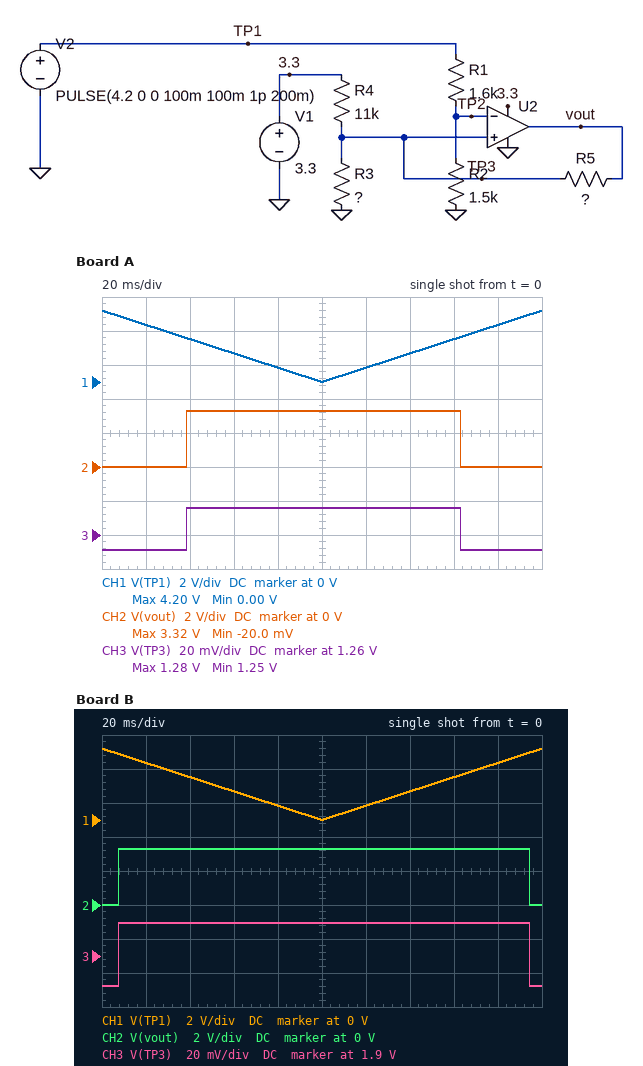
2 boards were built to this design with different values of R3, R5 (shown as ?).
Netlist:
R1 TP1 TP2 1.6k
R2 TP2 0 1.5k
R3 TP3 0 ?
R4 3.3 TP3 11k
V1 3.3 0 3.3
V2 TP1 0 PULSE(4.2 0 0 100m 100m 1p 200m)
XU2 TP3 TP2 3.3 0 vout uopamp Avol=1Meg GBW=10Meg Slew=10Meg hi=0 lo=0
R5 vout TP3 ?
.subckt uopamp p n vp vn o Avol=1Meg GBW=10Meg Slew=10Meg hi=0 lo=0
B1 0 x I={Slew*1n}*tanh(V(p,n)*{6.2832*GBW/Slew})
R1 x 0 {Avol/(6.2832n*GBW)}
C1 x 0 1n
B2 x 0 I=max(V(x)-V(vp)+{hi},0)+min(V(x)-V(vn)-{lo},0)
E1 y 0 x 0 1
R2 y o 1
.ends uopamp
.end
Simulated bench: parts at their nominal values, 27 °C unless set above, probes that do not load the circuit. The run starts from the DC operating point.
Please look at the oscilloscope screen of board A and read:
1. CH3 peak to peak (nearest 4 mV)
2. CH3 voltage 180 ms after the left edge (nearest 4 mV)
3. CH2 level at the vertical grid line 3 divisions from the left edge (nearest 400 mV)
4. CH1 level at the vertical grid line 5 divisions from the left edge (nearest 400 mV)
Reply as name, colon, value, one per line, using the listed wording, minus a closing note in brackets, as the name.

CH3 peak to peak: 24 mV
CH3 voltage 180 ms after the left edge: 1.252 V
CH2 level at the vertical grid line 3 divisions from the left edge: 3.2 V
CH1 level at the vertical grid line 5 divisions from the left edge: 0 V
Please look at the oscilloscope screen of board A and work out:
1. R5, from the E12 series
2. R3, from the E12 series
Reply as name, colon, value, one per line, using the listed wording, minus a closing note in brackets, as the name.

R5, from the E12 series: 560 kΩ
R3, from the E12 series: 6.8 kΩ
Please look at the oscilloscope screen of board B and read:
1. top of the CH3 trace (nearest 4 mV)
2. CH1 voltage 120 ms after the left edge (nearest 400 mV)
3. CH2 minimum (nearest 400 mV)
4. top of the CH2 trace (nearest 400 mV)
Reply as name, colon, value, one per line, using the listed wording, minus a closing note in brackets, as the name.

top of the CH3 trace: 1.920 V
CH1 voltage 120 ms after the left edge: 800 mV
CH2 minimum: 0 V
top of the CH2 trace: 3.2 V
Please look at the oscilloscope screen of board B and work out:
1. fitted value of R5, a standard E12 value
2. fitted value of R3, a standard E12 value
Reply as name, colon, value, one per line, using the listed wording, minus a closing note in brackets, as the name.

fitted value of R5, a standard E12 value: 560 kΩ
fitted value of R3, a standard E12 value: 15 kΩ
